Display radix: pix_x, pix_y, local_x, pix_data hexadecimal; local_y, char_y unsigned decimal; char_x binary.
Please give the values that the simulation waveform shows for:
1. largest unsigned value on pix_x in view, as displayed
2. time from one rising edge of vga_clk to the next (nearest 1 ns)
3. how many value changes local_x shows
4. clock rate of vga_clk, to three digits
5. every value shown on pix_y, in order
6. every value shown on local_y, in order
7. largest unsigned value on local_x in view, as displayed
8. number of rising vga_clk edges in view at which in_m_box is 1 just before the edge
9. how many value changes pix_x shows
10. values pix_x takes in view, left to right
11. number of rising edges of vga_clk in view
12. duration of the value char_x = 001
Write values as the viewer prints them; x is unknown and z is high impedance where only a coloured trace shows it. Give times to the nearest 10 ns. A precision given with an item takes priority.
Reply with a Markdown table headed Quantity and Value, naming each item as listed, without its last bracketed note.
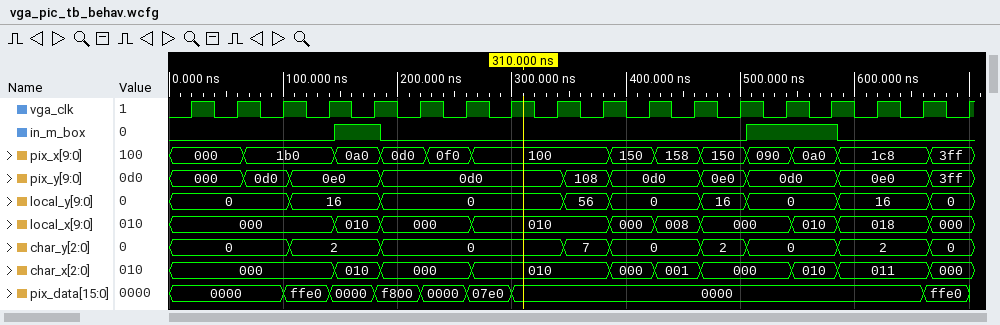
| Quantity | Value |
|---|---|
| largest unsigned value on pix_x in view, as displayed | 3ff |
| time from one rising edge of vga_clk to the next | 40 ns |
| how many value changes local_x shows | 9 |
| clock rate of vga_clk, to three digits | 25.0 MHz |
| every value shown on pix_y, in order | 000, 0d0, 0e0, 0d0, 108, 0d0, 0e0, 0d0, 0e0, 3ff |
| every value shown on local_y, in order | 0, 16, 0, 56, 0, 16, 0, 16, 0 |
| largest unsigned value on local_x in view, as displayed | 018 |
| number of rising vga_clk edges in view at which in_m_box is 1 just before the edge | 3 |
| how many value changes pix_x shows | 12 |
| values pix_x takes in view, left to right | 000, 1b0, 0a0, 0d0, 0f0, 100, 150, 158, 150, 090, 0a0, 1c8, 3ff |
| number of rising edges of vga_clk in view | 18 |
| duration of the value char_x = 001 | 40 ns |
